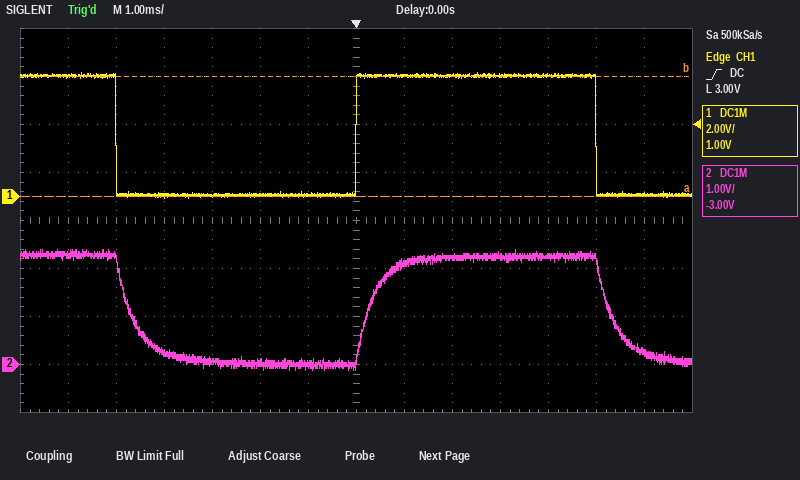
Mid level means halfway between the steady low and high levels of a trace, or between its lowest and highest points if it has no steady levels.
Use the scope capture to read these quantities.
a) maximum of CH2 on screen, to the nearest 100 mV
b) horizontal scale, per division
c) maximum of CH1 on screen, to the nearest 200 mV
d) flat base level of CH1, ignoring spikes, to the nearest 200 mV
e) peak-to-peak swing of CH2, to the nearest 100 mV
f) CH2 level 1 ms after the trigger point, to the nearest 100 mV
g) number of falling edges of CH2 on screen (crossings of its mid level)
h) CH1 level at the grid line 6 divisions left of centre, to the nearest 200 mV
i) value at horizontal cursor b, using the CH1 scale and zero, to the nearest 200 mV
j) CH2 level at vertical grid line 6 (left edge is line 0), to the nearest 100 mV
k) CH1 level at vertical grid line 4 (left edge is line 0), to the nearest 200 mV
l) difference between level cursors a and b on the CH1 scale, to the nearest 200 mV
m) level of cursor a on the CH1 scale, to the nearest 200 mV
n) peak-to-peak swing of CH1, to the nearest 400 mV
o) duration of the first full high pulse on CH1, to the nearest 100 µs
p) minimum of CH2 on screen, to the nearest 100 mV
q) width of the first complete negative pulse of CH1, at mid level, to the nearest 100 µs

2.4 V
1 ms
5.2 V
0.0 V
2.5 V
2.1 V
2
5.0 V
5.0 V
0.0 V
0.0 V
5.0 V
0.0 V
5.2 V
5.0 ms
-100 mV
5.0 ms
